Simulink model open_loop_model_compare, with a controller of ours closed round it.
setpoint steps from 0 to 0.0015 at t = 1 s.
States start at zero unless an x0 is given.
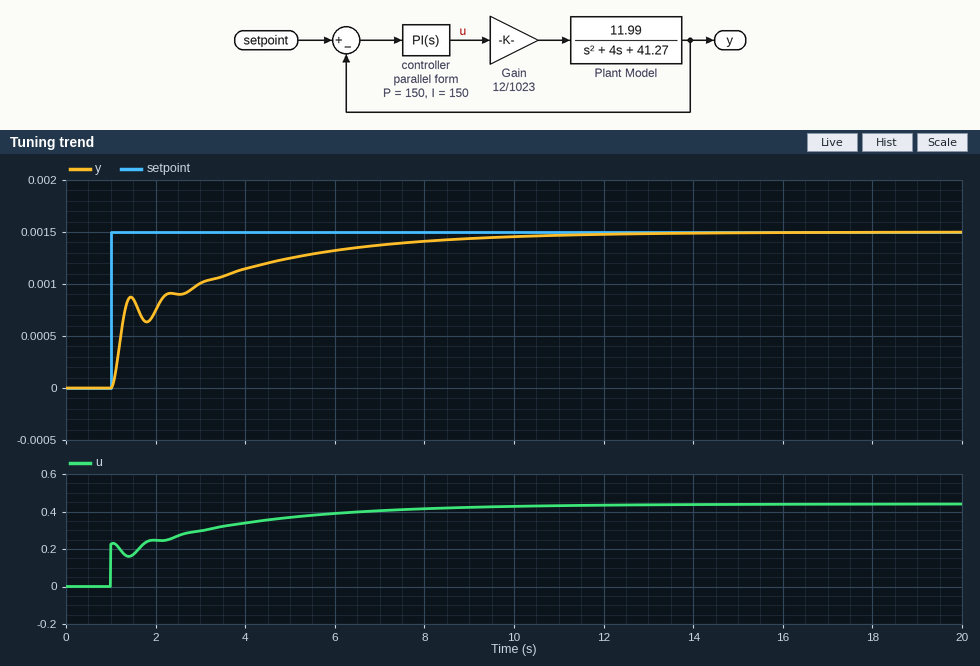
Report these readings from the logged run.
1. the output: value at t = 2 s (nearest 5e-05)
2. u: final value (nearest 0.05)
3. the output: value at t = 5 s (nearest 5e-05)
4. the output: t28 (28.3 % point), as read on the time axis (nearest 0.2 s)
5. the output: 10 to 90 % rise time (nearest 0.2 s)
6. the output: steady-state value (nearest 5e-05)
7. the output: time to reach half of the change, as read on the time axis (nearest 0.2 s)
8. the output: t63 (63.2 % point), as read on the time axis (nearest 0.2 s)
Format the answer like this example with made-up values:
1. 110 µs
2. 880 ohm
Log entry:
1. 0.00075
2. 0.45
3. 0.00125
4. 1.2 s
5. 5.4 s
6. 0.00150
7. 1.4 s
8. 2.8 s
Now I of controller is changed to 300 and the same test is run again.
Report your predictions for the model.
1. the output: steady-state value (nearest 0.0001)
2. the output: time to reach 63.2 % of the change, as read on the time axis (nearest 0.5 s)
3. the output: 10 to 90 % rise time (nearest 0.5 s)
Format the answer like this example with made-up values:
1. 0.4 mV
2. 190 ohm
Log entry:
1. 0.0015
2. 1.5 s
3. 2.5 s
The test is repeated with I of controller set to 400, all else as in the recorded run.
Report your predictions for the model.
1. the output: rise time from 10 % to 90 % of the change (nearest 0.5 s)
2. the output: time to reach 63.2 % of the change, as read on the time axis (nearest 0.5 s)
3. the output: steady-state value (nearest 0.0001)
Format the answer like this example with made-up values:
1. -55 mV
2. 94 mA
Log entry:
1. 2.0 s
2. 1.5 s
3. 0.0015
